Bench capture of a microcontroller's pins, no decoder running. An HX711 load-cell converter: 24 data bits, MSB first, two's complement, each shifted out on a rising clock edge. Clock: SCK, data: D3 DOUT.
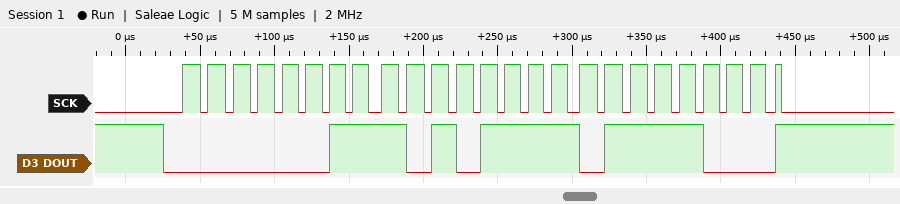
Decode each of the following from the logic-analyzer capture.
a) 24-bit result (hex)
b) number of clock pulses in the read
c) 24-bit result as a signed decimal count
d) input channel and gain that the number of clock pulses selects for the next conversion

0x03AF78
25
241528
channel A, gain 128
